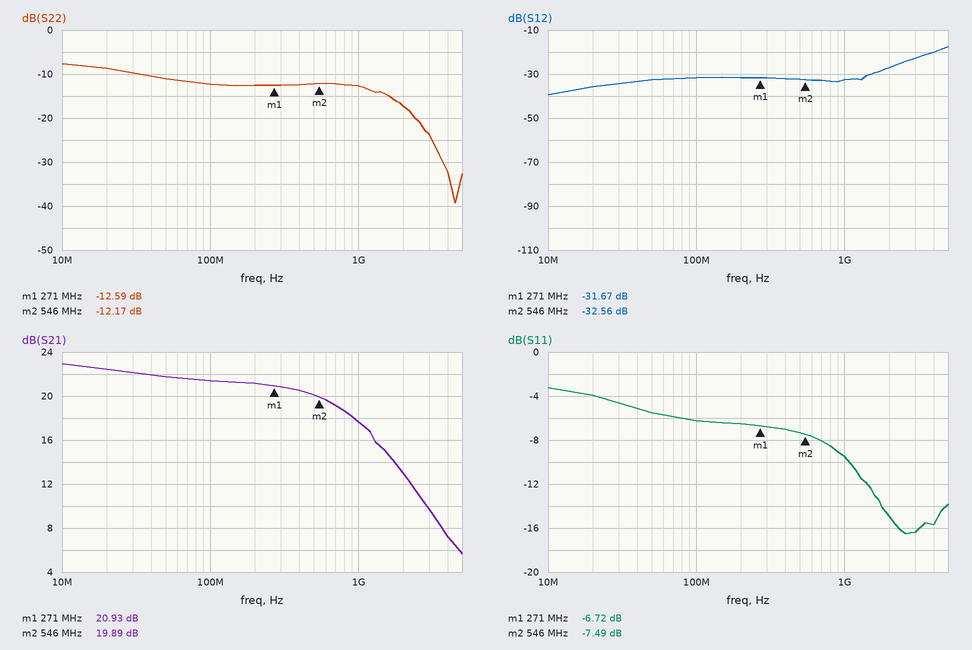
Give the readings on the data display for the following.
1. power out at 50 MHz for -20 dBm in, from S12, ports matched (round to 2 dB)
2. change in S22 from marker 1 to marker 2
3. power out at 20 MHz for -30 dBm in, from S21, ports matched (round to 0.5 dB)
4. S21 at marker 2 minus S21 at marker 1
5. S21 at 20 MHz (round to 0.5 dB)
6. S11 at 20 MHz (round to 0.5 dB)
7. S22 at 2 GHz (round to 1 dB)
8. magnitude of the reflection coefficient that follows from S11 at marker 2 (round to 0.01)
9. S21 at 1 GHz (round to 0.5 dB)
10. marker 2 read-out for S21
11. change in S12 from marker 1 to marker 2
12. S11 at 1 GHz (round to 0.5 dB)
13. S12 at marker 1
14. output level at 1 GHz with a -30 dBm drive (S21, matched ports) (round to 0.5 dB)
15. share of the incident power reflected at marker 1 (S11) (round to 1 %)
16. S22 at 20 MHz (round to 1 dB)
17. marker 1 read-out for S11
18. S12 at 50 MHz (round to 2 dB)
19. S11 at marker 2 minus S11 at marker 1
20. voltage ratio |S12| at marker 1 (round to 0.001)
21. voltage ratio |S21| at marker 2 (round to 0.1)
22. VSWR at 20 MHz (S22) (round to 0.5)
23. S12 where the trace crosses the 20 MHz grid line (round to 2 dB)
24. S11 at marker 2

-52 dBm
0.42 dB
-7.5 dBm
-1.04 dB
22.5 dB
-4.0 dB
-17 dB
0.42
17.5 dB
19.89 dB
-0.89 dB
-9.5 dB
-31.67 dB
-12.5 dBm
21 %
-9 dB
-6.72 dB
-32 dB
-0.77 dB
0.026
9.9
2.0
-36 dB
-7.49 dB
